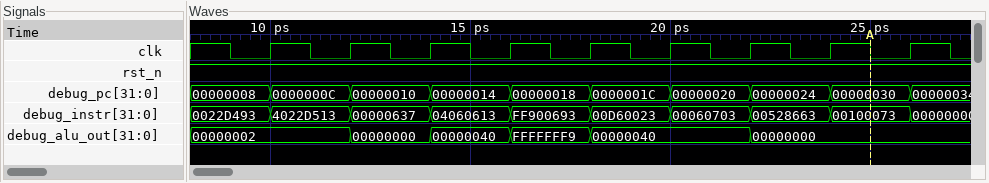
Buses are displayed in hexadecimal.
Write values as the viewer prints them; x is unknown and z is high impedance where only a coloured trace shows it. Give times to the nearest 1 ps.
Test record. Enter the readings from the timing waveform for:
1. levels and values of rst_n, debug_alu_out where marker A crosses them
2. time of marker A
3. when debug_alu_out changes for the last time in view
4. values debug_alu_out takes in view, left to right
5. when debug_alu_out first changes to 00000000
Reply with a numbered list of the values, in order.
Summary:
1. rst_n=1, debug_alu_out=00000000
2. 25 ps
3. 22 ps
4. 00000002, 00000000, 00000040, FFFFFFF9, 00000040, 00000000
5. 12 ps
